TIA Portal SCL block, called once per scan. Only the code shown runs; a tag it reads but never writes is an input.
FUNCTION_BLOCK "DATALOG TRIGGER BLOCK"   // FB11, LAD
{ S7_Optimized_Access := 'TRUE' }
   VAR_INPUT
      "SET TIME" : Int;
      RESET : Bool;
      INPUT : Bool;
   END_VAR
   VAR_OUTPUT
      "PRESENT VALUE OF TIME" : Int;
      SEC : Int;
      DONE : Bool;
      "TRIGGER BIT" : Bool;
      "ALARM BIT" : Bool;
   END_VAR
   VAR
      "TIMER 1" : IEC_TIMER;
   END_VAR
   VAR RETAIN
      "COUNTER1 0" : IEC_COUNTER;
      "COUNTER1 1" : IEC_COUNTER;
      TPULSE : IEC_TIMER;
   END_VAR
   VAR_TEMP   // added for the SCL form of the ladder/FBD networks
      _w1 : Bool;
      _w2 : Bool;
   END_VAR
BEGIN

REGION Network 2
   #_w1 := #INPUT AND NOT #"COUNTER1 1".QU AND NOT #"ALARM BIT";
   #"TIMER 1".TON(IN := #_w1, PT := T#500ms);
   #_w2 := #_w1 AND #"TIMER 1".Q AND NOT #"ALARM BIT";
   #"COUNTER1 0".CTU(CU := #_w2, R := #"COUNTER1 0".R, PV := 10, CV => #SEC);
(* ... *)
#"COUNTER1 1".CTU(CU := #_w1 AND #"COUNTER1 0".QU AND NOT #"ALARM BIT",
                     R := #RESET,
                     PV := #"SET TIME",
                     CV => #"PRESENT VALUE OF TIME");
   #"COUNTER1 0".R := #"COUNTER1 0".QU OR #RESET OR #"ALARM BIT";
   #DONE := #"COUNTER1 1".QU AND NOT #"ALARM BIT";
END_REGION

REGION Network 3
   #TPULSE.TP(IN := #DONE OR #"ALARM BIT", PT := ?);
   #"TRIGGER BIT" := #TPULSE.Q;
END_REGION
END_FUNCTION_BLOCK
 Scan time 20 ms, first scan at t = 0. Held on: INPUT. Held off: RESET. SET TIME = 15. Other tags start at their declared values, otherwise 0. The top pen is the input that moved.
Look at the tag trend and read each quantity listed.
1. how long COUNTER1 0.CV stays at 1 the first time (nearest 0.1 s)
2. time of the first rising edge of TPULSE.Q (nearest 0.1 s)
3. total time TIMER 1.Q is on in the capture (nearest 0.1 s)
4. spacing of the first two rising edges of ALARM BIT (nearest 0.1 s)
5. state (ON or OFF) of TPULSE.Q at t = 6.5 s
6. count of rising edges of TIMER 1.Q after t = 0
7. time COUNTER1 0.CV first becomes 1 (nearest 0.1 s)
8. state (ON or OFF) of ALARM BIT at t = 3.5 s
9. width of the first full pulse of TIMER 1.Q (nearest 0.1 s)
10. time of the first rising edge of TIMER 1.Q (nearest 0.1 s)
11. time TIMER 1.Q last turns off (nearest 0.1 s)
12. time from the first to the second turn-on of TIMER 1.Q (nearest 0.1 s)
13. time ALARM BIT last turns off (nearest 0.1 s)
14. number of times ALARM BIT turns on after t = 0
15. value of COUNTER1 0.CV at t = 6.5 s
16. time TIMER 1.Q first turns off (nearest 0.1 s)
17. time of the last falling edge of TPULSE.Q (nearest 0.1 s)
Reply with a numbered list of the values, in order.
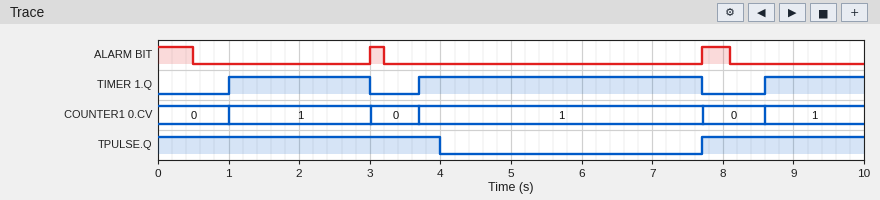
1. 2.0 s
2. 7.7 s
3. 7.4 s
4. 4.7 s
5. OFF
6. 3
7. 1.0 s
8. OFF
9. 2.0 s
10. 1.0 s
11. 7.7 s
12. 2.7 s
13. 8.1 s
14. 2
15. 1
16. 3.0 s
17. 4.0 s
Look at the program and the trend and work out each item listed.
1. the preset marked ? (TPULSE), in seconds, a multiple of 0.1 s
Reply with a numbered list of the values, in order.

1. 4.0 s
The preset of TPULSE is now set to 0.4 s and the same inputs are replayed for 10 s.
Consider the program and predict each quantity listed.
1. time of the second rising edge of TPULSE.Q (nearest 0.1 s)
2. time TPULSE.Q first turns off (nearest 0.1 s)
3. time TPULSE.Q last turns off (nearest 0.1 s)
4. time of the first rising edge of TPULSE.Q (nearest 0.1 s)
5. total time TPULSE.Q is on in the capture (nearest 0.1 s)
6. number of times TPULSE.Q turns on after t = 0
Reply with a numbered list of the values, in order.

1. 7.7 s
2. 0.4 s
3. 8.1 s
4. 3.0 s
5. 1.2 s
6. 2
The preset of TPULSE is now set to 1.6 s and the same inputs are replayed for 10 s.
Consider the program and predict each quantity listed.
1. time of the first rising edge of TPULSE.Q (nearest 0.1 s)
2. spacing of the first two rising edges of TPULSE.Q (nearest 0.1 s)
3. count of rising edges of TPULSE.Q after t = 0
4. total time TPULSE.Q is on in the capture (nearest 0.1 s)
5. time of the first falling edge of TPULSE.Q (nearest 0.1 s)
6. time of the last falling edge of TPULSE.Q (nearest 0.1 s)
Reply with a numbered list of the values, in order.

1. 3.0 s
2. 4.7 s
3. 2
4. 4.8 s
5. 1.6 s
6. 9.3 s
